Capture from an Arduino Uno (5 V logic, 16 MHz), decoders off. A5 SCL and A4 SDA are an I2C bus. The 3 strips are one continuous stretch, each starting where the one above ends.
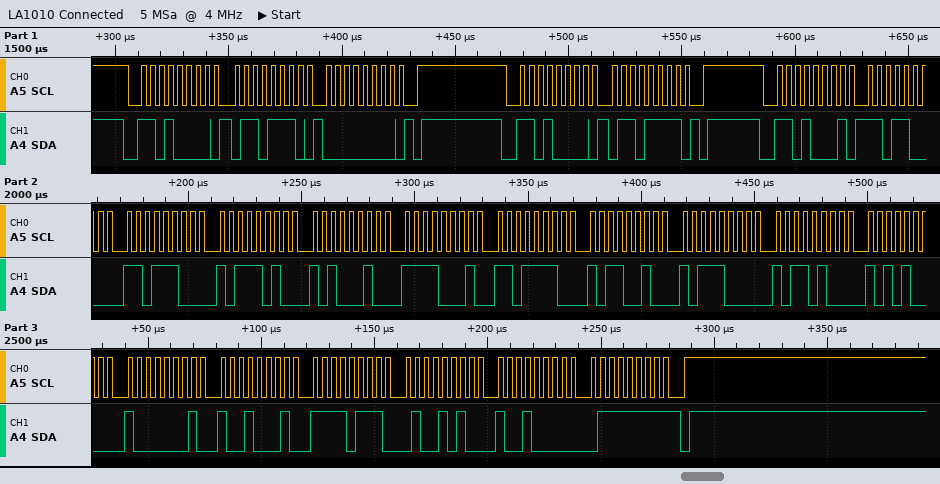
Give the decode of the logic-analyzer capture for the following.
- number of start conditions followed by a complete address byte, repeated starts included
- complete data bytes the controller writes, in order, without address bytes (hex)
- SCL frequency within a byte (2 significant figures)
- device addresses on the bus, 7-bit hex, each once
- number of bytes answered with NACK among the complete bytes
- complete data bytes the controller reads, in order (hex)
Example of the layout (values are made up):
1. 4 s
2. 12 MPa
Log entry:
1. 3
2. 6E 00 6F
3. 250 kHz
4. 0x68
5. 1
6. D8 DC BA A2 F1 DE B2 B8 B4 A8 81 91 F7 4A 90 7F
